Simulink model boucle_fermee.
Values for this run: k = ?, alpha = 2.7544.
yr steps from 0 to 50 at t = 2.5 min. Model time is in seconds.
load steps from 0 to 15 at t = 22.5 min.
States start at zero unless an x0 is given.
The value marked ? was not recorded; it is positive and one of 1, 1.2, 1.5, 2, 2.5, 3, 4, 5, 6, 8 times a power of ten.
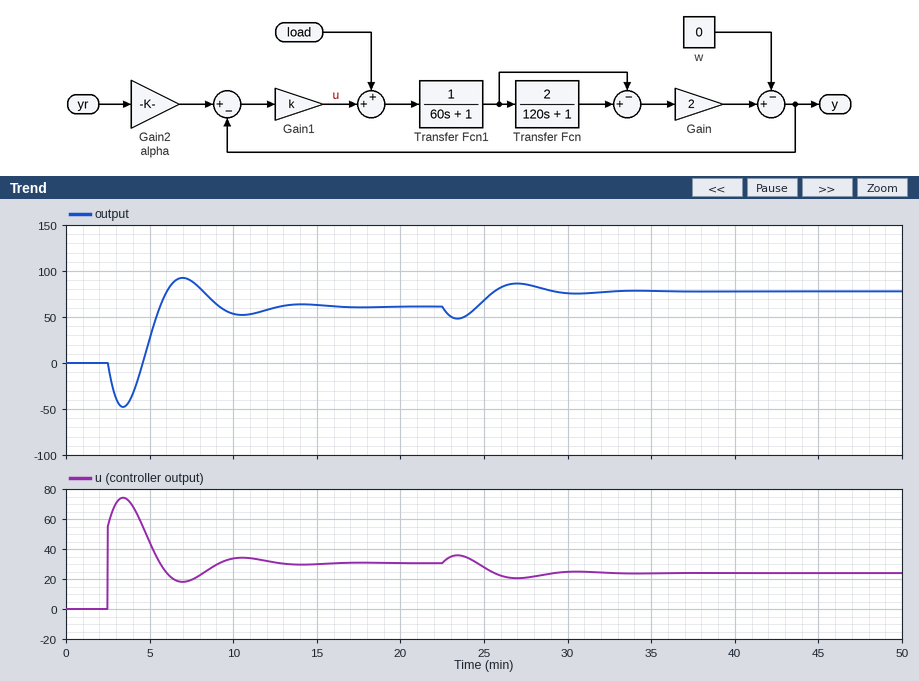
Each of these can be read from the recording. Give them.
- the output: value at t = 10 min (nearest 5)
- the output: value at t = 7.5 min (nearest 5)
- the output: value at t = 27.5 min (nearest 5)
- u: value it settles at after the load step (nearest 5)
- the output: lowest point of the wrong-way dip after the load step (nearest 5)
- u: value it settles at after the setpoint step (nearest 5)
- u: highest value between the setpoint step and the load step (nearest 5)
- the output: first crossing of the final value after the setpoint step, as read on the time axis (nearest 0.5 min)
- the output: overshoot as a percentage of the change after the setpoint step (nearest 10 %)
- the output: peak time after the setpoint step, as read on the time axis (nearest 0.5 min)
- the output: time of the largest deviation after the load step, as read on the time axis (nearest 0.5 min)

55
90
85
25
50
30
75
5.5 min
50 %
7.0 min
27.0 min
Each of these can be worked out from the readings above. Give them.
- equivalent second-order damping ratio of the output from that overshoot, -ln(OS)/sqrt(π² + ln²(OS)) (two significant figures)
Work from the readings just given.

0.22
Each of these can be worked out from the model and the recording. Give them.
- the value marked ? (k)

0.4
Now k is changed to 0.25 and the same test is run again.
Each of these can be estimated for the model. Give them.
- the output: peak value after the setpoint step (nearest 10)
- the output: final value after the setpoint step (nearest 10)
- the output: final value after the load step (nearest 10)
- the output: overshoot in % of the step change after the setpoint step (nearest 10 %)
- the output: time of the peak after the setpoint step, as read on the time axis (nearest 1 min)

50
50
70
20 %
8 min
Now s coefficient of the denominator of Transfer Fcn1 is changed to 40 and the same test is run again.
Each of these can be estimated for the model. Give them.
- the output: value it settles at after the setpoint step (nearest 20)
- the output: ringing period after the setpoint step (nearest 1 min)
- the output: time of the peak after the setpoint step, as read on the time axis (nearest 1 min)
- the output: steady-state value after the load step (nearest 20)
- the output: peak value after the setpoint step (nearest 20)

60
6 min
6 min
80
100
